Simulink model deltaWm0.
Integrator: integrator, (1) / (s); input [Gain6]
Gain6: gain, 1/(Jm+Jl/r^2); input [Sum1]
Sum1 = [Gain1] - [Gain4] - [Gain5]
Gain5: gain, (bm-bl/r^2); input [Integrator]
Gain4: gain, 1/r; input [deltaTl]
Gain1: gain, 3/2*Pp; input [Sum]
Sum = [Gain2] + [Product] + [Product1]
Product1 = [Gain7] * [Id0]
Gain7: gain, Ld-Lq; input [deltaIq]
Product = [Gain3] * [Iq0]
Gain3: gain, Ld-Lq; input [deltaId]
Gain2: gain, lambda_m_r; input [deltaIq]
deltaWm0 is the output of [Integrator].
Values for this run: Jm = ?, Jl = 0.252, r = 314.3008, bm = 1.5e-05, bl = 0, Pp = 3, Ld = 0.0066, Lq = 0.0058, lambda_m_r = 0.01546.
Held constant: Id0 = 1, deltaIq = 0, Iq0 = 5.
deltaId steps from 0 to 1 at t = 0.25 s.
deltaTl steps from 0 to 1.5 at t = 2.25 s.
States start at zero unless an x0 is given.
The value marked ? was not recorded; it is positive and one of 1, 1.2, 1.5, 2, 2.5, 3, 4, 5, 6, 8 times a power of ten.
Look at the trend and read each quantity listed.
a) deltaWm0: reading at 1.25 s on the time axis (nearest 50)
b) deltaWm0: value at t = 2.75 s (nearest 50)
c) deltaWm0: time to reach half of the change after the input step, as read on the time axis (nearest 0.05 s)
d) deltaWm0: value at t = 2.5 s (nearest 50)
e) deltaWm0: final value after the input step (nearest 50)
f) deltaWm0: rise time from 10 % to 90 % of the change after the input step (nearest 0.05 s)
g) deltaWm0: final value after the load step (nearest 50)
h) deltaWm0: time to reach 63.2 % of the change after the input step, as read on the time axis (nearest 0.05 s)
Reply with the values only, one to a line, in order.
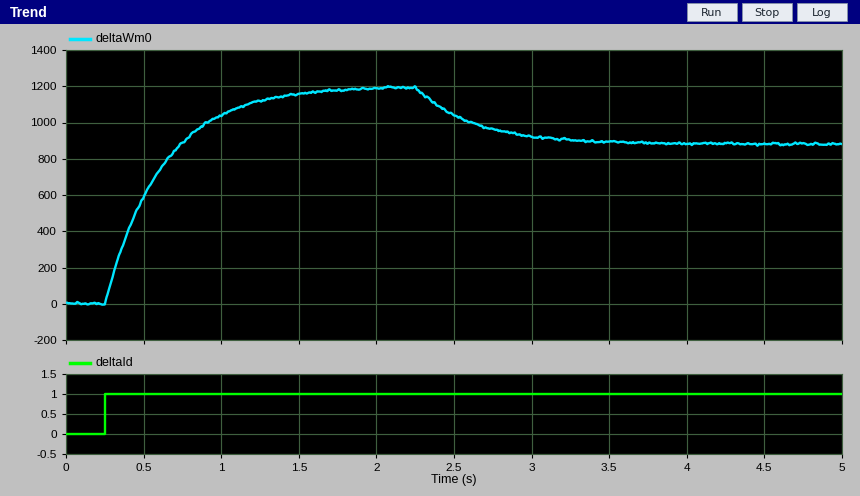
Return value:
1100
950
0.50 s
1050
1200
0.80 s
900
0.60 s
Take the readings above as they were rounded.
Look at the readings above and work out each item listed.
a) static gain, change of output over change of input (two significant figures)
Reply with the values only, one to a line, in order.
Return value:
1200
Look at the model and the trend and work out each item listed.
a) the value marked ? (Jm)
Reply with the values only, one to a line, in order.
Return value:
3e-06
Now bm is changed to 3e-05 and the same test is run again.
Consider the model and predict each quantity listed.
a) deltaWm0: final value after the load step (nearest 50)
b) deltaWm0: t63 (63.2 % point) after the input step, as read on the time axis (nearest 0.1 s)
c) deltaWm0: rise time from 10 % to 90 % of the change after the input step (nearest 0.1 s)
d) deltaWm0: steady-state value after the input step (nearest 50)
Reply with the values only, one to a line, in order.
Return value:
450
0.4 s
0.4 s
600
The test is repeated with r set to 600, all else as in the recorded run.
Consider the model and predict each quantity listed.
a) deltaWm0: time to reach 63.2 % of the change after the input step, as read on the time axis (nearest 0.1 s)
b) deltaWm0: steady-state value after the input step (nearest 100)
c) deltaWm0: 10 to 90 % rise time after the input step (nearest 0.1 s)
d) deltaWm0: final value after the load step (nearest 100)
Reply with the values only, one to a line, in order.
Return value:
0.5 s
1200
0.5 s
1000
